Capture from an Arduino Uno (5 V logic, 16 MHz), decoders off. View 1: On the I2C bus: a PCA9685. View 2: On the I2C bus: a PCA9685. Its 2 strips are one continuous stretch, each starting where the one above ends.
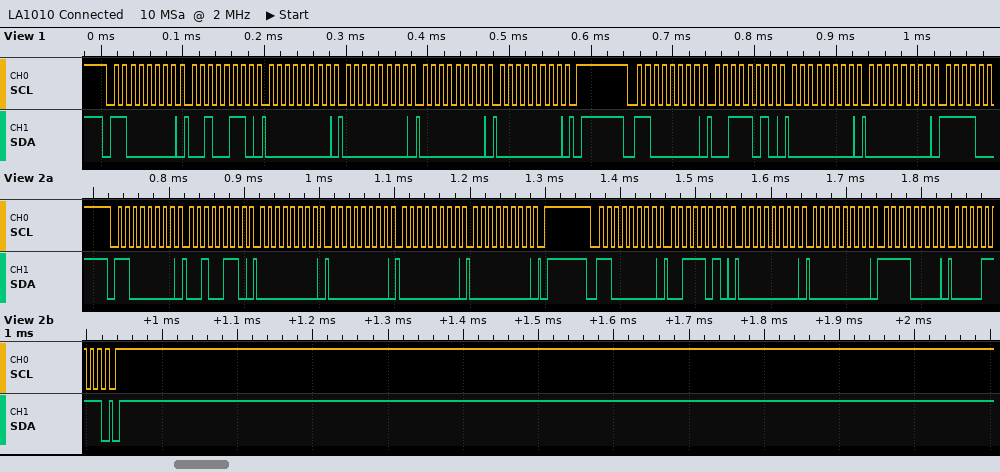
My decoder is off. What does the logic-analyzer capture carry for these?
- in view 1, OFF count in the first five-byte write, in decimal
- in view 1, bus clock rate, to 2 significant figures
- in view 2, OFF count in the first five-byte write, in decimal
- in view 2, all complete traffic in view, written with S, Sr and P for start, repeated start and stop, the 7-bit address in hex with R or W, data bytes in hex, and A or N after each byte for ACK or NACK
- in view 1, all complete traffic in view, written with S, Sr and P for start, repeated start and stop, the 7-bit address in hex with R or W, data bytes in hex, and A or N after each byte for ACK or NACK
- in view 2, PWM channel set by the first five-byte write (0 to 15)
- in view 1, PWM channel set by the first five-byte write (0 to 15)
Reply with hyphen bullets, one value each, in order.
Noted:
- 0
- 100 kHz
- 0
- S 60W A 26 A 00 A 00 A 00 A 00 A P S 60W A 3A A 00 A 00 A F0 A 0F A P
- S 60W A 26 A 00 A 00 A 00 A 00 A P S 60W A 3A A 00 A 00 A
- 8
- 8
